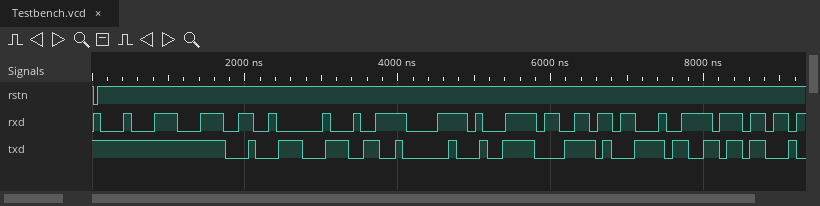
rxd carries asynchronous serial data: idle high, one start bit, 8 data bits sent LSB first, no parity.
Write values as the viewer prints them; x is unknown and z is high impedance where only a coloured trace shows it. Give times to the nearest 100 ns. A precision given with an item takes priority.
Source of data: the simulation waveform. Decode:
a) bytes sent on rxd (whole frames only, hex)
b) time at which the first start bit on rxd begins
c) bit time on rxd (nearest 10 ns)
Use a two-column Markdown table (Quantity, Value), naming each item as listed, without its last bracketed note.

| Quantity | Value |
|---|---|
| bytes sent on rxd | C4, 9C, 02, E4, 78, BC, B6, E4, B7 |
| time at which the first start bit on rxd begins | 100 ns |
| bit time on rxd | 100 ns |
